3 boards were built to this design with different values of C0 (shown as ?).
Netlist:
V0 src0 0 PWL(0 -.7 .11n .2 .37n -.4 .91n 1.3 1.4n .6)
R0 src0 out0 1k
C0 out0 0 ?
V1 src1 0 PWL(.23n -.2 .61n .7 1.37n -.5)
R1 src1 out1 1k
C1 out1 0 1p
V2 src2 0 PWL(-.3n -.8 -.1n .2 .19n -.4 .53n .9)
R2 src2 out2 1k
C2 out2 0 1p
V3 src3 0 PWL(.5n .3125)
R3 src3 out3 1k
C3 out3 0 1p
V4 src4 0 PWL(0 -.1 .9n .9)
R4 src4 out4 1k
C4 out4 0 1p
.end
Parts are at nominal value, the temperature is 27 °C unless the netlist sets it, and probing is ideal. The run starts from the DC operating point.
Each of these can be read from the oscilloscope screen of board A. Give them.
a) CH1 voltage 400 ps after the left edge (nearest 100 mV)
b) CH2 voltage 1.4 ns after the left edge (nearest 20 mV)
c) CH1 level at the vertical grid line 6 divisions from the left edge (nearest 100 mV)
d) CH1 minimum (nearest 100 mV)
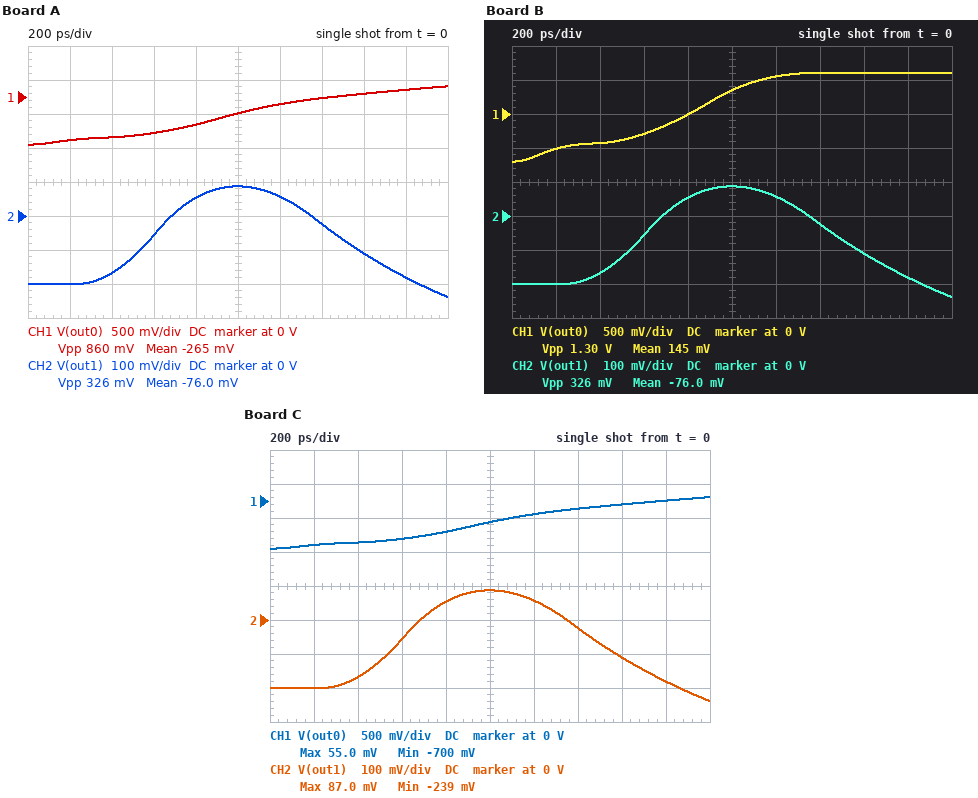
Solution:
-600 mV
-20 mV
-100 mV
-700 mV
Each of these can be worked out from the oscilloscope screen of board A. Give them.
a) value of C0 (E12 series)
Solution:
1.8 pF
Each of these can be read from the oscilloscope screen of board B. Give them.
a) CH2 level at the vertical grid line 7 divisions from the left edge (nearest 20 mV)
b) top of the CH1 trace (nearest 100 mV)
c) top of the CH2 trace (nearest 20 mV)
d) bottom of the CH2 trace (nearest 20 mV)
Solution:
-20 mV
600 mV
80 mV
-240 mV
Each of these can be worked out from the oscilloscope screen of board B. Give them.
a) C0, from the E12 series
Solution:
560 fF
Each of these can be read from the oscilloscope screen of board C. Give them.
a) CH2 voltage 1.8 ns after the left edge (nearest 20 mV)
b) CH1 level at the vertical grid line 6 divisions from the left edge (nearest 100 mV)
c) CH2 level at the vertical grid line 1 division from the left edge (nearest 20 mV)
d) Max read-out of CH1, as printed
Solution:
-180 mV
-200 mV
-200 mV
55.0 mV
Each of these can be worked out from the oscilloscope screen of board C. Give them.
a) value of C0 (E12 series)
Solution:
2.2 pF
